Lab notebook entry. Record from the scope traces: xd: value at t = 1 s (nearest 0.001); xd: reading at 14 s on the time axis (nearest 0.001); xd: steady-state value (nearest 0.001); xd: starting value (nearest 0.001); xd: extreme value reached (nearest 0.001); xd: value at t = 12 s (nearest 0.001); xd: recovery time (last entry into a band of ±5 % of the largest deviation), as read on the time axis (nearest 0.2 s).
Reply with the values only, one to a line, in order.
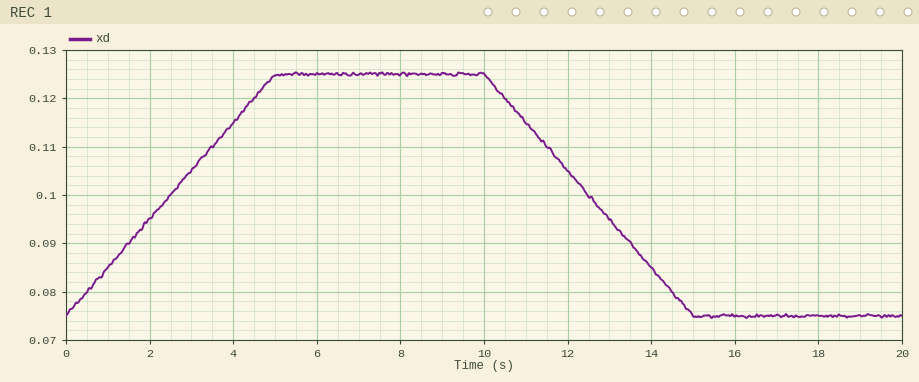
0.085
0.085
0.075
0.075
0.125
0.105
14.8 s
